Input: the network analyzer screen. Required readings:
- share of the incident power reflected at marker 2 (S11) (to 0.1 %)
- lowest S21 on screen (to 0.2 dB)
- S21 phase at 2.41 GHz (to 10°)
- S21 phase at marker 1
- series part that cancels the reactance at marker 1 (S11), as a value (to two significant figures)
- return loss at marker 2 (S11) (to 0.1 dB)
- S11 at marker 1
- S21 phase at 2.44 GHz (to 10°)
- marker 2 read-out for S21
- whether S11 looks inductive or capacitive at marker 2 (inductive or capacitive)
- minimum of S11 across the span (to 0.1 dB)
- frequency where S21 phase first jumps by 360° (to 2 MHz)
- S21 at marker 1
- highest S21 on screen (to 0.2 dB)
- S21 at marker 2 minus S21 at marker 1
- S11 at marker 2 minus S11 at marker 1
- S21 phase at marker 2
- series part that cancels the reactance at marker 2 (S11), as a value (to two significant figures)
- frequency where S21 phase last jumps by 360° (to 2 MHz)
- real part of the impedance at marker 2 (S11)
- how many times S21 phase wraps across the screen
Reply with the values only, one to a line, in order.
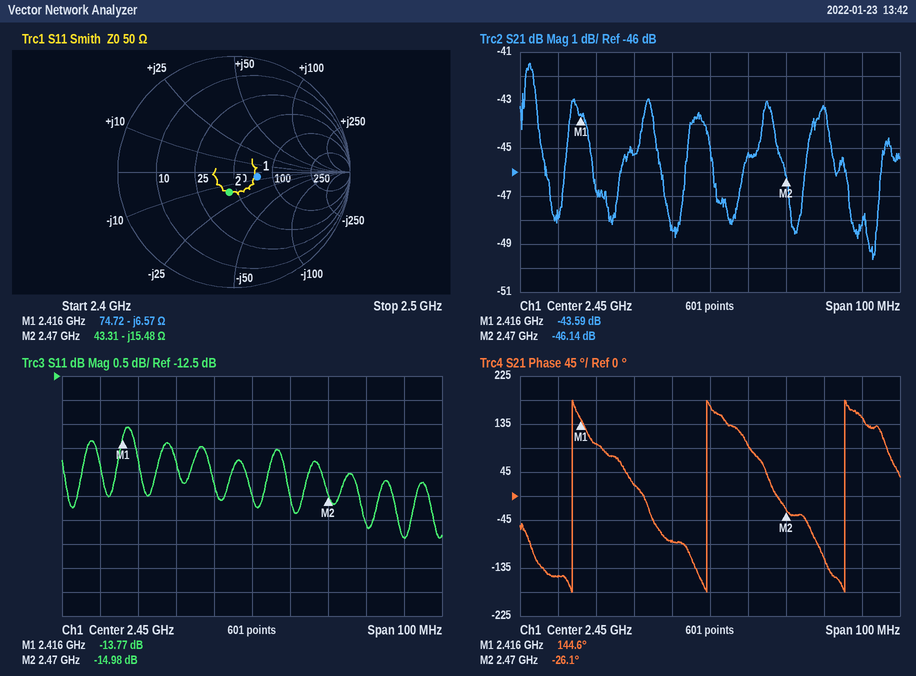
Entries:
3.2 %
-49.6 dB
-150°
144.6°
430 pH
15.0 dB
-13.77 dB
-80°
-46.14 dB
capacitive
-15.9 dB
2.414 GHz
-43.59 dB
-41.4 dB
-2.55 dB
-1.21 dB
-26.1°
1.00 nH
2.486 GHz
43.31 Ω
3
